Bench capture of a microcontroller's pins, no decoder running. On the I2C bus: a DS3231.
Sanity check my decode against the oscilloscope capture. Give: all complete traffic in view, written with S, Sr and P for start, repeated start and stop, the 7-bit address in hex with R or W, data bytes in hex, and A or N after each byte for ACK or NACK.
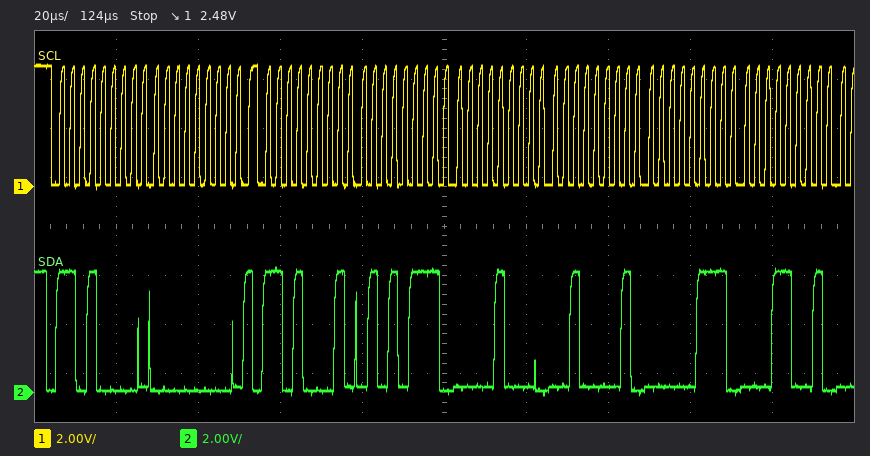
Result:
S 68W A 00 A Sr 68R A 57 A 08 A 21 A 07 A 19 A
